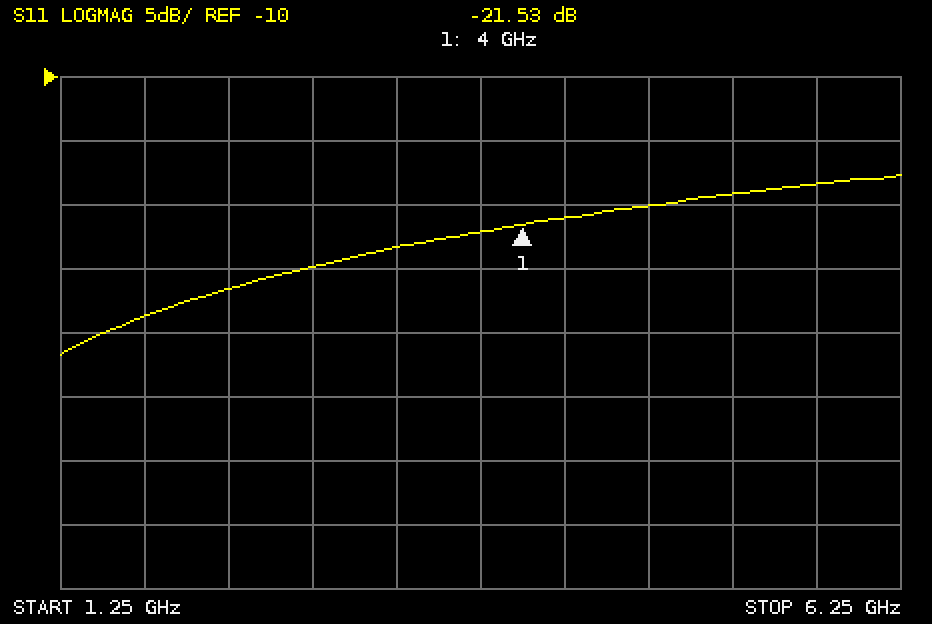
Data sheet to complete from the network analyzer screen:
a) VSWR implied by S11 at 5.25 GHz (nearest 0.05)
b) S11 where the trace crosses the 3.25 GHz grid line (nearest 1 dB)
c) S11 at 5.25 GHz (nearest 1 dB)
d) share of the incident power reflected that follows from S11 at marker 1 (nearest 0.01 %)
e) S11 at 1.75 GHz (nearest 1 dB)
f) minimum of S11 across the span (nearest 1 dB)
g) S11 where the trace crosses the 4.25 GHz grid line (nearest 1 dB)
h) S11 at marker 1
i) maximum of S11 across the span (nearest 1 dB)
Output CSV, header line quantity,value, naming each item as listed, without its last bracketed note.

quantity,value
VSWR implied by S11 at 5.25 GHz,1.25
S11 where the trace crosses the 3.25 GHz grid line,-23 dB
S11 at 5.25 GHz,-19 dB
share of the incident power reflected that follows from S11 at marker 1,0.70 %
S11 at 1.75 GHz,-29 dB
minimum of S11 across the span,-32 dB
S11 where the trace crosses the 4.25 GHz grid line,-21 dB
S11 at marker 1,-21.53 dB
maximum of S11 across the span,-18 dB
